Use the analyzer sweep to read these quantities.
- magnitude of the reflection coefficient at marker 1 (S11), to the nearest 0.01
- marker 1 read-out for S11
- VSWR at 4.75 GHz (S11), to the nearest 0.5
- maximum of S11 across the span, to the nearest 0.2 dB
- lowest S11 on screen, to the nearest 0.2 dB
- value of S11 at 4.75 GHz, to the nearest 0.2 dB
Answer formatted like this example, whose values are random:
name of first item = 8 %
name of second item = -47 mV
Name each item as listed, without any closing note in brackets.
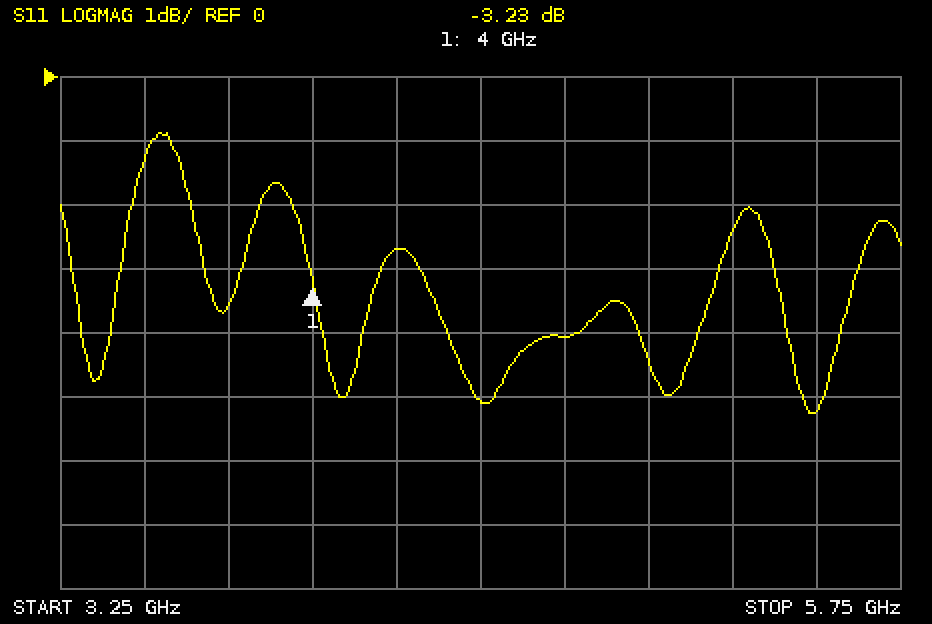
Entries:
magnitude of the reflection coefficient at marker 1 (S11), to the nearest 0.01 = 0.69
marker 1 read-out for S11 = -3.23 dB
VSWR at 4.75 GHz (S11), to the nearest 0.5 = 4.5
maximum of S11 across the span, to the nearest 0.2 dB = -0.8 dB
lowest S11 on screen, to the nearest 0.2 dB = -5.2 dB
value of S11 at 4.75 GHz, to the nearest 0.2 dB = -4.0 dB
